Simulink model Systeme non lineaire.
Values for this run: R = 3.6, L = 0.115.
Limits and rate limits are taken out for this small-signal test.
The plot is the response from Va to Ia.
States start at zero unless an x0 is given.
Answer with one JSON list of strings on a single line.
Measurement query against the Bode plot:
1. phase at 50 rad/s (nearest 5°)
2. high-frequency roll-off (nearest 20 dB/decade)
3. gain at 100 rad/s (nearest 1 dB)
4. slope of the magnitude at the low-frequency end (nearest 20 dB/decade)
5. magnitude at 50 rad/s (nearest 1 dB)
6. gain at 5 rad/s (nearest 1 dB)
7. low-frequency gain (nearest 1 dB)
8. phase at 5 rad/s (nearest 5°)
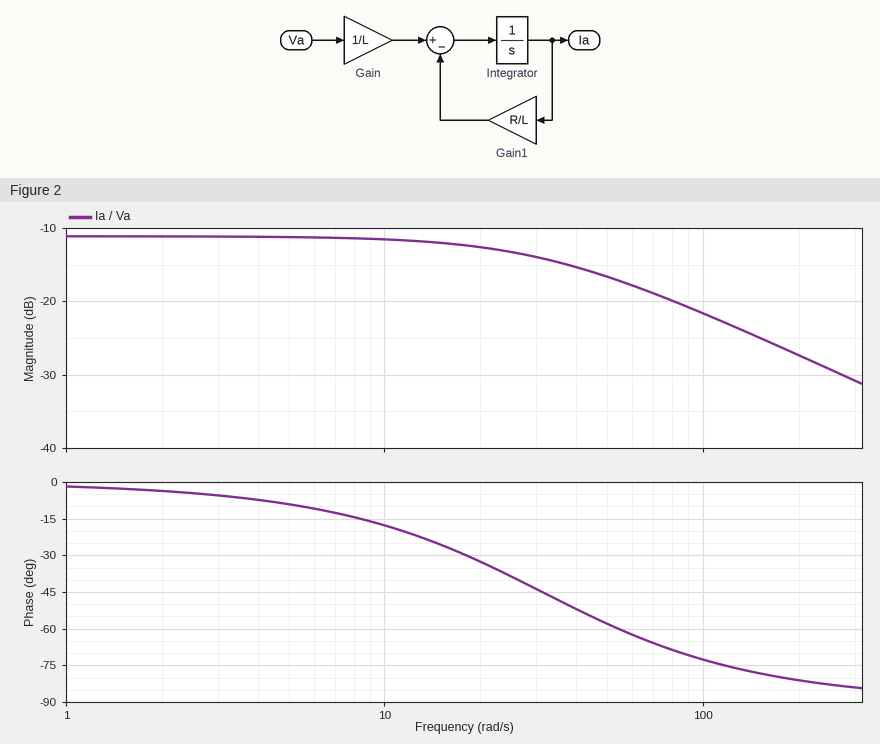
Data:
["-60°", "-20 dB/decade", "-22 dB", "0 dB/decade", "-17 dB", "-11 dB", "-11 dB", "-10°"]
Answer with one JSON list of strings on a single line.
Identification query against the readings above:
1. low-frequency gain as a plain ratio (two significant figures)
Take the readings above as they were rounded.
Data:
["0.28"]
